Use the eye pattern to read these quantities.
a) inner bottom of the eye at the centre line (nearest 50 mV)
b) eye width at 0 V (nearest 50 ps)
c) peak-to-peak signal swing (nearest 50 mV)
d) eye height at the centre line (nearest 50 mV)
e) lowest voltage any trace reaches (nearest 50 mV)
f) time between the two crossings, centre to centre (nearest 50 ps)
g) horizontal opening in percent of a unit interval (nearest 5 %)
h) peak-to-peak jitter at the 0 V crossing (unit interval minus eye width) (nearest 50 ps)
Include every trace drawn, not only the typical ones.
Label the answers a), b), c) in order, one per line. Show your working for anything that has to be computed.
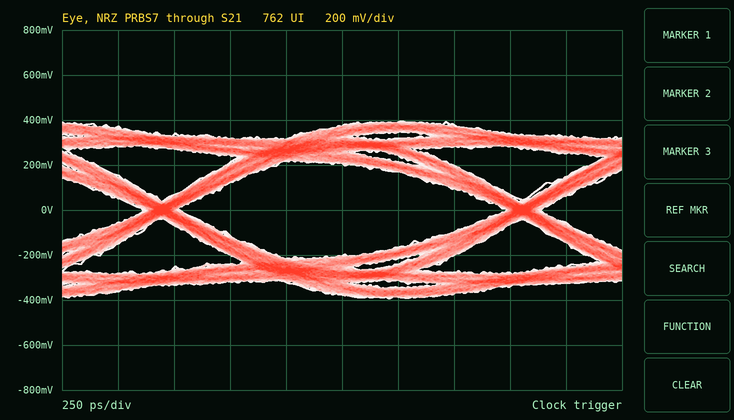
a) -200 mV
b) 1.45 ns
c) 800 mV
d) 400 mV
e) -400 mV
f) 1.60 ns
g) 1.45 ns / 1.60 ns ≈ 90.6 %, so 90 % to the nearest 5 %
h) 150 ps
